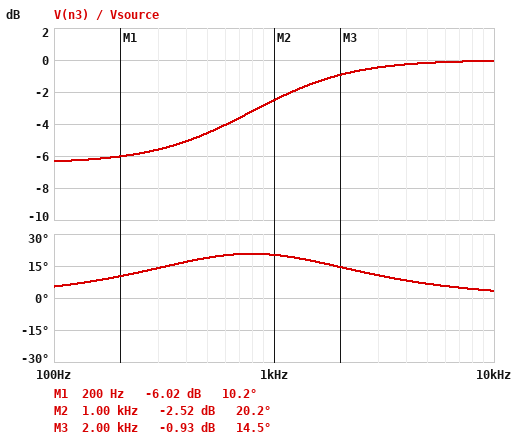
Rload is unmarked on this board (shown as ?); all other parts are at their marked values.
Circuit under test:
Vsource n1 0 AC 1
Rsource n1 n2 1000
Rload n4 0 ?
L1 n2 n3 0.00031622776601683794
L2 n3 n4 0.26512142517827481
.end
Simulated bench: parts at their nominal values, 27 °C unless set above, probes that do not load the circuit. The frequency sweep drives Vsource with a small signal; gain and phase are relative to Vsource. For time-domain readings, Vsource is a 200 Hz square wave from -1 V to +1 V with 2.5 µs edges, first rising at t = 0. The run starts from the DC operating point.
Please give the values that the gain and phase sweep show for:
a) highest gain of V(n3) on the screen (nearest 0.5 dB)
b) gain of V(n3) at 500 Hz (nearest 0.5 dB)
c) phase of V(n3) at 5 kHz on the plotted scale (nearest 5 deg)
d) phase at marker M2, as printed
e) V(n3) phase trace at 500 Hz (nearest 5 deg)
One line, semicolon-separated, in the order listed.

0 dB; -4.5 dB; 5 deg; 20.2 deg; 20 deg
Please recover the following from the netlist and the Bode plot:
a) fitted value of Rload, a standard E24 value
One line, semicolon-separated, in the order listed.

910 Ω
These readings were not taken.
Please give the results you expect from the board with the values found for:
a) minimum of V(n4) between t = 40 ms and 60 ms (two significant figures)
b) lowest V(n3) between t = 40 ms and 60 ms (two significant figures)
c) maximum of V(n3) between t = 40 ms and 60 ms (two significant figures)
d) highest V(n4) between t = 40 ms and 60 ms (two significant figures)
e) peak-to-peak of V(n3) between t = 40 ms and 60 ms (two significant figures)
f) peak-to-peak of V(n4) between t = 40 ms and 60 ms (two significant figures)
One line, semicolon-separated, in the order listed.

-480 mV; -1.5 V; 1.5 V; 480 mV; 3.0 V; 950 mV
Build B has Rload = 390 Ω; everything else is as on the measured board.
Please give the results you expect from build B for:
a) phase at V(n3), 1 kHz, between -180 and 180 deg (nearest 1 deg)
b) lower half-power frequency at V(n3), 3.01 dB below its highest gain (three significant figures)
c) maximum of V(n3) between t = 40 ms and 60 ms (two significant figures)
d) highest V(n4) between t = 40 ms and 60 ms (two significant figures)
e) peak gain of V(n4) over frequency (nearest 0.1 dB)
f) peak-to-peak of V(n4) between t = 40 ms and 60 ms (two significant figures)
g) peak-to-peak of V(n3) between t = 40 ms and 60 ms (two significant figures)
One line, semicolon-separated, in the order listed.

27 deg; 765 Hz; 1.7 V; 280 mV; -11.0 dB; 560 mV; 3.4 V
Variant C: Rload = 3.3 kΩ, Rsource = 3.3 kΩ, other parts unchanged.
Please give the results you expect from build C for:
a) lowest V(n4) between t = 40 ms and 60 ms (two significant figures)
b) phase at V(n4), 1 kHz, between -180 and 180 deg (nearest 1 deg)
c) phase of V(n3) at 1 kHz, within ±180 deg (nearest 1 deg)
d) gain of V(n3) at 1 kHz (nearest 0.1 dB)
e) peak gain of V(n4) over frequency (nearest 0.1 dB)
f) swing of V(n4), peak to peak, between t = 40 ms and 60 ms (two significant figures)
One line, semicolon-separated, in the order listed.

-500 mV; -14 deg; 13 deg; -5.3 dB; -6.0 dB; 1.0 V
